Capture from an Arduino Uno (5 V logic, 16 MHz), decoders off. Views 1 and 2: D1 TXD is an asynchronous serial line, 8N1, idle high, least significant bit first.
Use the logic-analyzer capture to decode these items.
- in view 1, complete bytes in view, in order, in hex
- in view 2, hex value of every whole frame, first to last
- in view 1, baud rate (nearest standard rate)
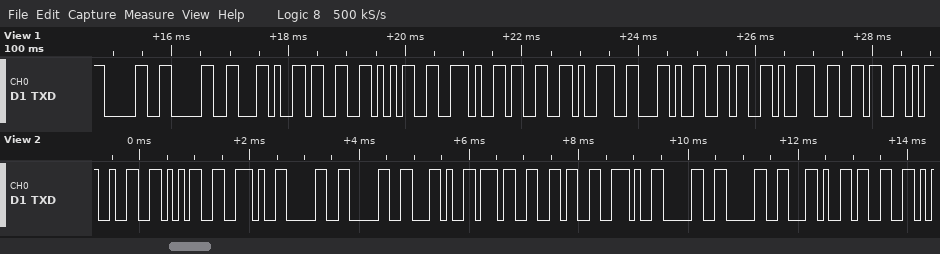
30 30 2C 33 35 2E 33 39 2C 36 39 36
32 35 2E 30 30 2C 37 36 2E 30 30 2C 33
9600 baud
